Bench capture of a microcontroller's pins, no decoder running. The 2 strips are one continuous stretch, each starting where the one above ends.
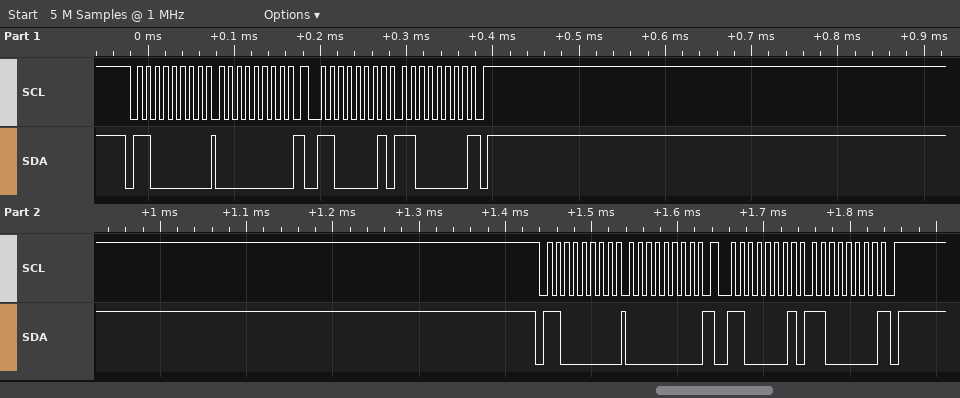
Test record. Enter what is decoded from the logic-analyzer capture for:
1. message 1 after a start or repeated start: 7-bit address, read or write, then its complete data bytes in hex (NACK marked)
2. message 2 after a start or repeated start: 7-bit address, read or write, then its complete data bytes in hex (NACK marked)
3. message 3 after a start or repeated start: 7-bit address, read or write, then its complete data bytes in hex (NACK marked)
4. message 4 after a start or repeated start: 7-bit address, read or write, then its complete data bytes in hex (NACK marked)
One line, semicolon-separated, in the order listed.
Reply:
0x60 write: 00; 0x60 read: C0 NACK; 0x60 write: 00; 0x60 read: C0 NACK
